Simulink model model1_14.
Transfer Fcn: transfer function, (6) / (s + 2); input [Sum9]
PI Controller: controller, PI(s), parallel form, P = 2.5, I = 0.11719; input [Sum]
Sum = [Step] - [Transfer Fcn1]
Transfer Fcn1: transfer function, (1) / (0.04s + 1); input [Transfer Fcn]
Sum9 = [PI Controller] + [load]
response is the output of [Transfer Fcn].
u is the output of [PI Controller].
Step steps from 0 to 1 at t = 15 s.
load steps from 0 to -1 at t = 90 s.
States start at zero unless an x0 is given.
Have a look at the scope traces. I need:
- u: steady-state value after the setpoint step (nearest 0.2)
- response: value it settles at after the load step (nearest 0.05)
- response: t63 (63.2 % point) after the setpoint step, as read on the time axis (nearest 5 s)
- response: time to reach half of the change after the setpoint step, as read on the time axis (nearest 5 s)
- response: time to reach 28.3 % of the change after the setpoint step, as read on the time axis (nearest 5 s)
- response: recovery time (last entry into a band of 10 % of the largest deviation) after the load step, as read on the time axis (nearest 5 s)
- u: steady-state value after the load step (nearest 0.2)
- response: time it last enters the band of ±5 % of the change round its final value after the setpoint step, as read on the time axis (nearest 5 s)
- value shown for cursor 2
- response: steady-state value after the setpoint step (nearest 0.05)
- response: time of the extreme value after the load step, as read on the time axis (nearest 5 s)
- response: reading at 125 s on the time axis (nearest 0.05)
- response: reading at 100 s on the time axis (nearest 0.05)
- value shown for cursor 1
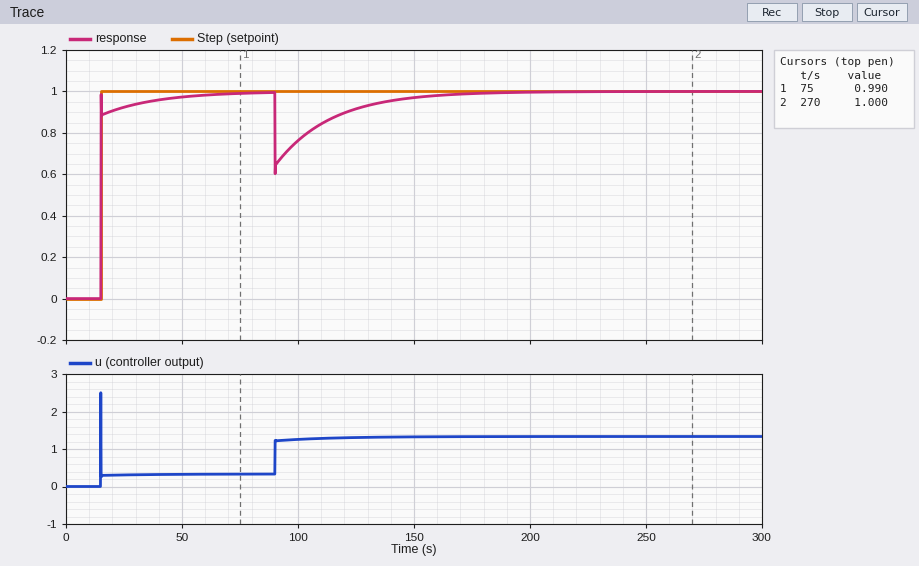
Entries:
0.4
1.00
15 s
15 s
15 s
145 s
1.4
35 s
1.000
1.00
90 s
0.90
0.75
0.990
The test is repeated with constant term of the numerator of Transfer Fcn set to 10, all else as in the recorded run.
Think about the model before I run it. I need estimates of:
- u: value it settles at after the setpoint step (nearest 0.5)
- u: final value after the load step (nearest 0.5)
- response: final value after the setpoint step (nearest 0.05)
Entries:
0.0
1.0
1.00
